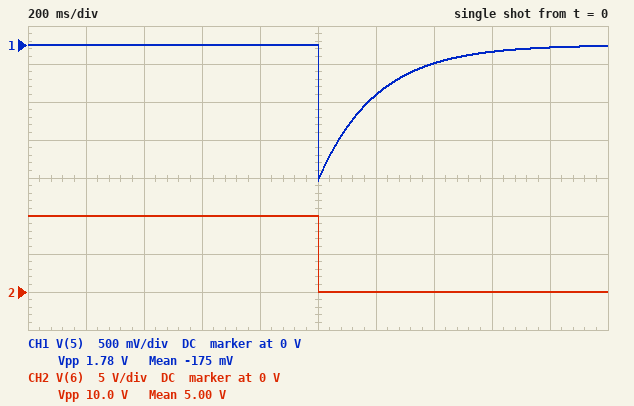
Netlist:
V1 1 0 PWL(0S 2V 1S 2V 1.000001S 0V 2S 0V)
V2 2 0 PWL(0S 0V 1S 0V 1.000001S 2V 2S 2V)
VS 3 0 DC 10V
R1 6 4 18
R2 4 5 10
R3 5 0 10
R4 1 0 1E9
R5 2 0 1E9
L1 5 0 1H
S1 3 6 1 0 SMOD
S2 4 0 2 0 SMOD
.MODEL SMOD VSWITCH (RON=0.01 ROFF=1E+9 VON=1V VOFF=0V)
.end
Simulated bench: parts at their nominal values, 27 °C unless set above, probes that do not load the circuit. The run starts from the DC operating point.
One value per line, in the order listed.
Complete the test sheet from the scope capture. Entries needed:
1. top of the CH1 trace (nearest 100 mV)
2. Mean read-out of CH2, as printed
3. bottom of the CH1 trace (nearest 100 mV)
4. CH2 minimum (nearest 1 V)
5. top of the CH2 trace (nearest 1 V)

0 V
5.00 V
-1.8 V
0 V
10 V
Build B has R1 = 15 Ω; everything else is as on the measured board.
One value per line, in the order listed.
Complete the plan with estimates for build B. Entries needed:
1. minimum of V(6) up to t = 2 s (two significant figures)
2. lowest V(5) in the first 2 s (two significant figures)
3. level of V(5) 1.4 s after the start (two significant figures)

-2.0 mV
-2.0 V
-270 mV
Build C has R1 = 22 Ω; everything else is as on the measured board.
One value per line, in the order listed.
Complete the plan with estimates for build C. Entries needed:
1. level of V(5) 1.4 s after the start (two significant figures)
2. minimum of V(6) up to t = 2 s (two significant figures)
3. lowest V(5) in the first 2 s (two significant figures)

-210 mV
-1.6 mV
-1.6 V
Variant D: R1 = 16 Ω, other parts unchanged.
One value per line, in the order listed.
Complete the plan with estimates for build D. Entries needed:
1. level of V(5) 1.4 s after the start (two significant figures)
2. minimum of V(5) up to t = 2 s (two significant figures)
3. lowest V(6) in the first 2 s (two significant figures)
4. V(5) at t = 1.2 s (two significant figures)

-260 mV
-1.9 V
-1.9 mV
-710 mV
